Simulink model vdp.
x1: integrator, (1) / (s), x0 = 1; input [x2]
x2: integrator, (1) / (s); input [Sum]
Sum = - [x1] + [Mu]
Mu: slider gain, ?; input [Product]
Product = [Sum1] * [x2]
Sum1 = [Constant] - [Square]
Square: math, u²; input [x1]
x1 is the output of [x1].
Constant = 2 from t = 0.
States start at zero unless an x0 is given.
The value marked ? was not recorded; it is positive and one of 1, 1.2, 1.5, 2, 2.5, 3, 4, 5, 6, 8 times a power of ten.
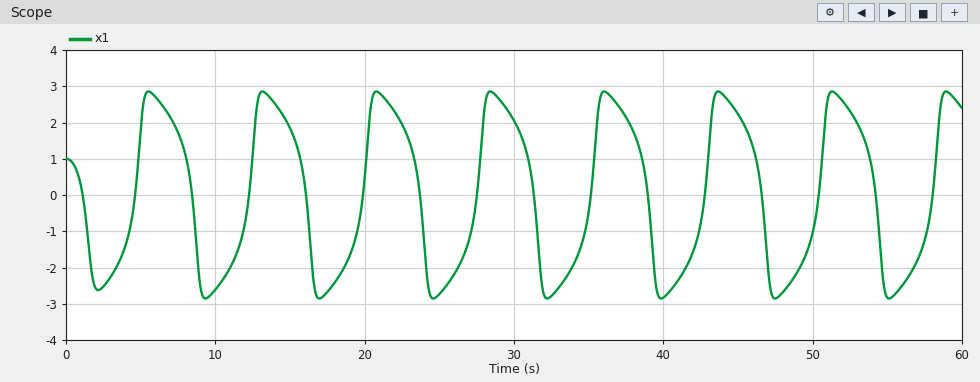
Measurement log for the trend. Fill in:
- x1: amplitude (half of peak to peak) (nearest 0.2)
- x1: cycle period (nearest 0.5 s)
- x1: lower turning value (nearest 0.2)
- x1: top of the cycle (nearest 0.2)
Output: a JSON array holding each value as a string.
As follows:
["2.8", "7.5 s", "-2.8", "2.8"]
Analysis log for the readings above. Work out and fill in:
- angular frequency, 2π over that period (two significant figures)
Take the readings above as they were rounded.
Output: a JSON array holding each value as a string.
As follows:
["0.84 rad/s"]
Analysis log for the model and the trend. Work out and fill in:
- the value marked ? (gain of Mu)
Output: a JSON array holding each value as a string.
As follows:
["1"]
